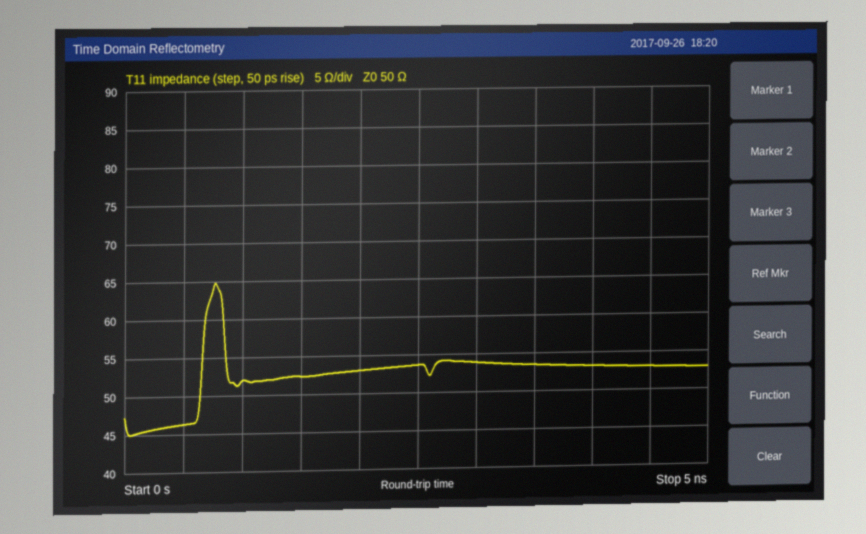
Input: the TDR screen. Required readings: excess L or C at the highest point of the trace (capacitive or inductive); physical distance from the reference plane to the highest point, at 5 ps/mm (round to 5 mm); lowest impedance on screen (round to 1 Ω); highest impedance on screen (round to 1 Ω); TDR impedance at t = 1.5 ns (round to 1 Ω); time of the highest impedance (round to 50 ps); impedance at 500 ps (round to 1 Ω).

inductive
75 mm
45 Ω
65 Ω
52 Ω
750 ps
46 Ω
